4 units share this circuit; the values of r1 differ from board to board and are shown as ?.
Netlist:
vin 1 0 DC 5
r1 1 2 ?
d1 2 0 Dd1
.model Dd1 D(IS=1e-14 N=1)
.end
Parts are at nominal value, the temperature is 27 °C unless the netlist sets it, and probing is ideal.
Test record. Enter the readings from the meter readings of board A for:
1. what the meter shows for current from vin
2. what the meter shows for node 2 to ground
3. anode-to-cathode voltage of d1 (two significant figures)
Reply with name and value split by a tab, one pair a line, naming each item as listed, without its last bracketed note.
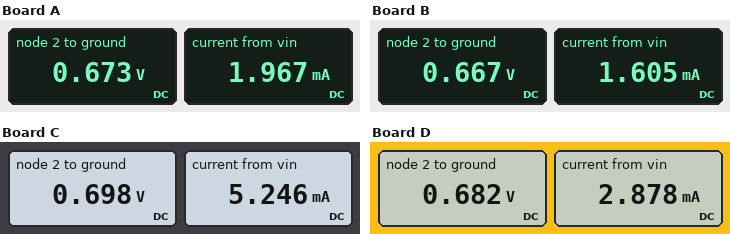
what the meter shows for current from vin	1.967 mA
what the meter shows for node 2 to ground	0.673 V
anode-to-cathode voltage of d1	670 mV
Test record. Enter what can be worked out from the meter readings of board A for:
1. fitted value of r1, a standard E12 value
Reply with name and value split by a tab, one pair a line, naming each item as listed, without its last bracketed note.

fitted value of r1, a standard E12 value	2.2 kΩ
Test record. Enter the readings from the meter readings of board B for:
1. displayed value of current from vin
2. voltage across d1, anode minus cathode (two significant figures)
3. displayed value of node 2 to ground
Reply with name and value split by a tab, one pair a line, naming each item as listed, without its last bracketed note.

displayed value of current from vin	1.605 mA
voltage across d1, anode minus cathode	670 mV
displayed value of node 2 to ground	0.667 V
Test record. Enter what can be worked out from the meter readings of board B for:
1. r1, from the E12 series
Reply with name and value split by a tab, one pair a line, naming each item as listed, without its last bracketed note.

r1, from the E12 series	2.7 kΩ
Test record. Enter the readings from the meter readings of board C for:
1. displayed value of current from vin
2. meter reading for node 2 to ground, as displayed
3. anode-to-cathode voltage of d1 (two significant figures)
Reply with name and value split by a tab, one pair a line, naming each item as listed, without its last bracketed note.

displayed value of current from vin	5.246 mA
meter reading for node 2 to ground, as displayed	0.698 V
anode-to-cathode voltage of d1	700 mV
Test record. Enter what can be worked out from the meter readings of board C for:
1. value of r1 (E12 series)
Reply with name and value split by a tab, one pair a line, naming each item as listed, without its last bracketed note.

value of r1	820 Ω
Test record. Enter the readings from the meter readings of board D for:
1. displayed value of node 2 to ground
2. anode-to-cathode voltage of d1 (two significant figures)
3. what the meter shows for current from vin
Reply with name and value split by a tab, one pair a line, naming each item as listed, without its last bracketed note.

displayed value of node 2 to ground	0.682 V
anode-to-cathode voltage of d1	680 mV
what the meter shows for current from vin	2.878 mA
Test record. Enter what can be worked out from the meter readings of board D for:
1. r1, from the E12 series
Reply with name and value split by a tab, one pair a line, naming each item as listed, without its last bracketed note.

r1, from the E12 series	1.5 kΩ
